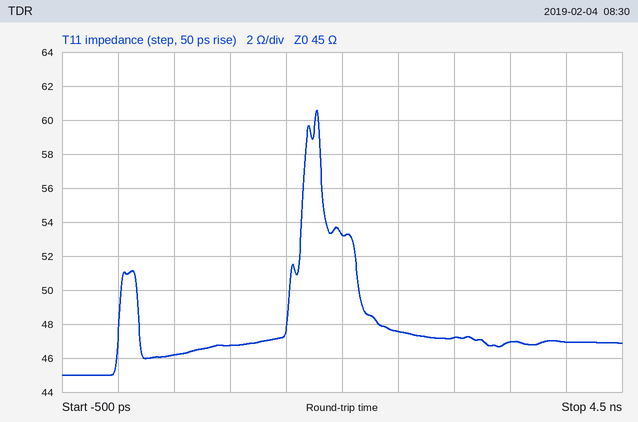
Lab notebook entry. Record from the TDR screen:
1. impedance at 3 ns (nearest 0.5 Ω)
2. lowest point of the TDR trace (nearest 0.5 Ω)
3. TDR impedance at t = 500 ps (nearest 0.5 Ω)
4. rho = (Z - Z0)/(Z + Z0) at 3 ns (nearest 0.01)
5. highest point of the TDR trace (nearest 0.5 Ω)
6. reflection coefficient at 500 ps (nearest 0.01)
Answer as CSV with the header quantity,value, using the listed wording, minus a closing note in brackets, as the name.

quantity,value
impedance at 3 ns,47.0 Ω
lowest point of the TDR trace,45.0 Ω
TDR impedance at t = 500 ps,46.0 Ω
rho = (Z - Z0)/(Z + Z0) at 3 ns,+0.02
highest point of the TDR trace,60.5 Ω
reflection coefficient at 500 ps,+0.01
